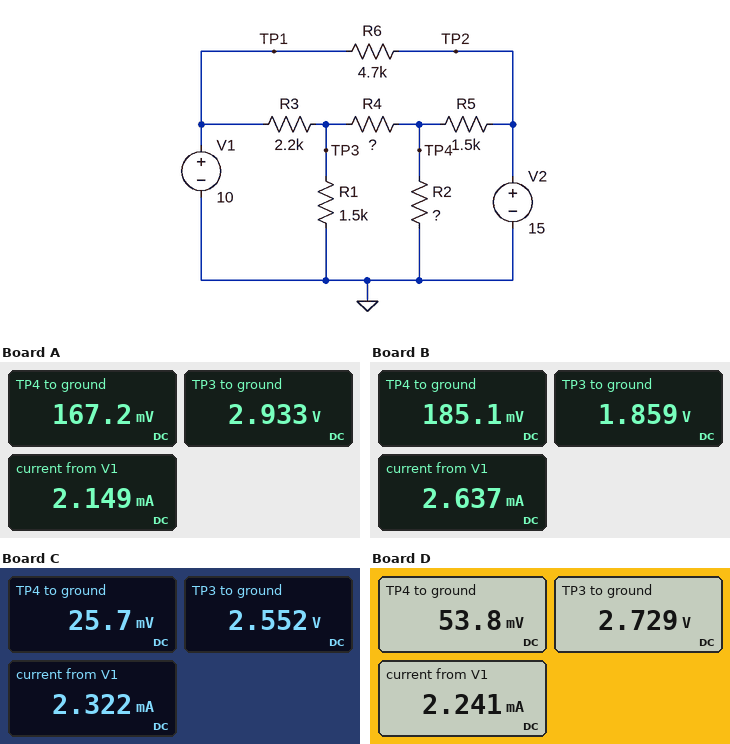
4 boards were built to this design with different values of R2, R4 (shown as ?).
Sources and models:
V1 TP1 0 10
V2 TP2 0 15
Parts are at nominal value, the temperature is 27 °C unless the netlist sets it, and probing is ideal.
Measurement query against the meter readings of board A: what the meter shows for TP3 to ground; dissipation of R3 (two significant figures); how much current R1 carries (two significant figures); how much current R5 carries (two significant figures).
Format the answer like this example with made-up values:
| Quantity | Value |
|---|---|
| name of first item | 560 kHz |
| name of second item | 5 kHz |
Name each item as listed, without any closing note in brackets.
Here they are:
| Quantity | Value |
|---|---|
| what the meter shows for TP3 to ground | 2.933 V |
| dissipation of R3 | 23 mW |
| how much current R1 carries | 2.0 mA |
| how much current R5 carries | 9.9 mA |
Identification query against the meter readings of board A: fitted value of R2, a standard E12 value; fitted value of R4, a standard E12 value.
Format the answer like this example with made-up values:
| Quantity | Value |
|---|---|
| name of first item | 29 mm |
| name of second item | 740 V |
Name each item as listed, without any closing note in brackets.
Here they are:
| Quantity | Value |
|---|---|
| fitted value of R2, a standard E12 value | 15 Ω |
| fitted value of R4, a standard E12 value | 2.2 kΩ |
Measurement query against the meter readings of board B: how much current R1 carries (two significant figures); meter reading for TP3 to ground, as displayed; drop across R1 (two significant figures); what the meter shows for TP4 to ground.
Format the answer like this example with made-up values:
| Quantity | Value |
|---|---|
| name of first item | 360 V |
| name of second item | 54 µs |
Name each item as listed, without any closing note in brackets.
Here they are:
| Quantity | Value |
|---|---|
| how much current R1 carries | 1.2 mA |
| meter reading for TP3 to ground, as displayed | 1.859 V |
| drop across R1 | 1.9 V |
| what the meter shows for TP4 to ground | 185.1 mV |
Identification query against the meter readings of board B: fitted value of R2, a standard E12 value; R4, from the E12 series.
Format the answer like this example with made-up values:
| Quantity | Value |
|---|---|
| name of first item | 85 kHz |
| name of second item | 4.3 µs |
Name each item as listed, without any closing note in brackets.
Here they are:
| Quantity | Value |
|---|---|
| fitted value of R2, a standard E12 value | 15 Ω |
| R4, from the E12 series | 680 Ω |
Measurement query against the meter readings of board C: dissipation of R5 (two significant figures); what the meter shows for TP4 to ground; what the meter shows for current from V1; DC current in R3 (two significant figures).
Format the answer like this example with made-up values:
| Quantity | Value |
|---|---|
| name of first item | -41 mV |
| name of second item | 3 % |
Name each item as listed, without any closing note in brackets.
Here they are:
| Quantity | Value |
|---|---|
| dissipation of R5 | 150 mW |
| what the meter shows for TP4 to ground | 25.7 mV |
| what the meter shows for current from V1 | 2.322 mA |
| DC current in R3 | 3.4 mA |
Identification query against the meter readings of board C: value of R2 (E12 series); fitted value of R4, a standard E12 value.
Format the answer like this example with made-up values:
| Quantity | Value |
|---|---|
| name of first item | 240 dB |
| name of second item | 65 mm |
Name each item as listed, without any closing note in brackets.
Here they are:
| Quantity | Value |
|---|---|
| value of R2 | 2.2 Ω |
| fitted value of R4, a standard E12 value | 1.5 kΩ |
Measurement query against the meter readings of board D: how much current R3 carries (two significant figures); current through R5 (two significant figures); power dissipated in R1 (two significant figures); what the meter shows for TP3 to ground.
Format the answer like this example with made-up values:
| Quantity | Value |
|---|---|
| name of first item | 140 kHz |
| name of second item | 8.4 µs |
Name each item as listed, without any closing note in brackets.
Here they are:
| Quantity | Value |
|---|---|
| how much current R3 carries | 3.3 mA |
| current through R5 | 10 mA |
| power dissipated in R1 | 5.0 mW |
| what the meter shows for TP3 to ground | 2.729 V |
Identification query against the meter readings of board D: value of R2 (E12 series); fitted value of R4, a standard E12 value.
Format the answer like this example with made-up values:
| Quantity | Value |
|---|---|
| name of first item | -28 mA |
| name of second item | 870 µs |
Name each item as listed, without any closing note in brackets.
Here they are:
| Quantity | Value |
|---|---|
| value of R2 | 4.7 Ω |
| fitted value of R4, a standard E12 value | 1.8 kΩ |
